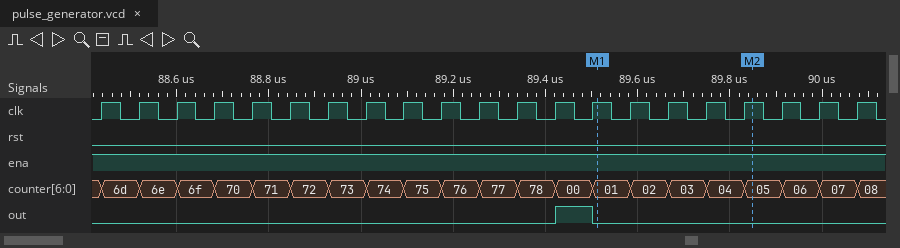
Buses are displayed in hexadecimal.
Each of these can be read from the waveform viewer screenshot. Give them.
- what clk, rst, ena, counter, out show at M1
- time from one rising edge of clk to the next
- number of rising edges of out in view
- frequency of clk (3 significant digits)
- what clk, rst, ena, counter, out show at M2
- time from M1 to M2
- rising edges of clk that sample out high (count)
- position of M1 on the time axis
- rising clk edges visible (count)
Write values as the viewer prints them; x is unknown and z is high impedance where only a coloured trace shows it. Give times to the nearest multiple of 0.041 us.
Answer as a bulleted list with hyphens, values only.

- clk=1, rst=0, ena=1, counter=01, out=0
- 0.082 us
- 1
- 12.2 MHz
- clk=1, rst=0, ena=1, counter=05, out=0
- 0.328 us
- 1
- 89.503 us
- 21
